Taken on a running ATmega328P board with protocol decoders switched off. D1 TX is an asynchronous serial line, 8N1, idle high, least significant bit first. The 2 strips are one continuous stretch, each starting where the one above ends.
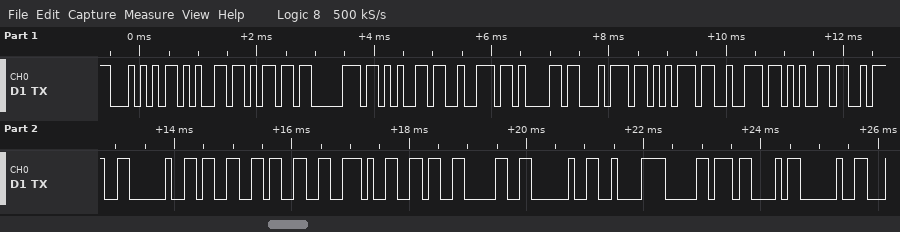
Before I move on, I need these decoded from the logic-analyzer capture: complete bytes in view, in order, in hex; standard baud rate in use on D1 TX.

54 65 6D 70 65 72 61 74 75 72 65 3A 20 33 33 2E 36 30 20 C2 B0 43 20
9600 baud
